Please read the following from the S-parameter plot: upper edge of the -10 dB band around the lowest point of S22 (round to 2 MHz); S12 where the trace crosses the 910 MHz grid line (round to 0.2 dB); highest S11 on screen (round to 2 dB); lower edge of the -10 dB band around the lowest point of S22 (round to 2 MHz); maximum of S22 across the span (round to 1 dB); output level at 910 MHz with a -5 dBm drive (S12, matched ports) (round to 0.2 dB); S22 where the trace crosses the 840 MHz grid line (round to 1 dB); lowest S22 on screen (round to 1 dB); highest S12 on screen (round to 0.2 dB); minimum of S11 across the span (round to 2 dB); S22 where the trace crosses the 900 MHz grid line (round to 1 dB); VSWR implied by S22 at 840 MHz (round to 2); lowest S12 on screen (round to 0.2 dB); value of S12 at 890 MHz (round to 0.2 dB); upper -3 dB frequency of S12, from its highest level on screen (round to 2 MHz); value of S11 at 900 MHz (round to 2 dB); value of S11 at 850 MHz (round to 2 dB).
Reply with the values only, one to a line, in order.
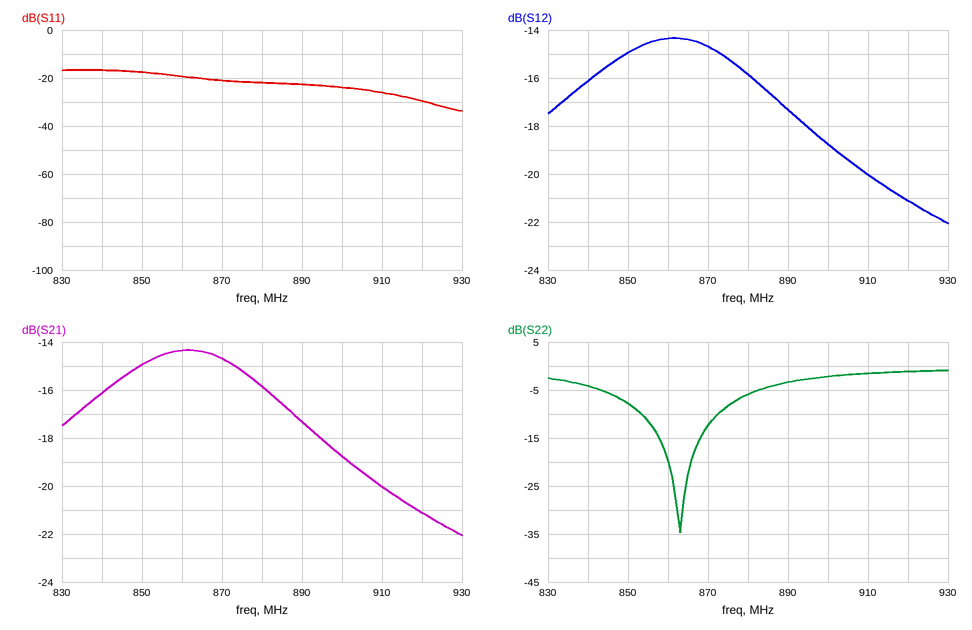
872 MHz
-20.0 dB
-16 dB
854 MHz
-1 dB
-25.0 dBm
-4 dB
-35 dB
-14.4 dB
-34 dB
-2 dB
4
-22.0 dB
-17.4 dB
890 MHz
-24 dB
-18 dB
